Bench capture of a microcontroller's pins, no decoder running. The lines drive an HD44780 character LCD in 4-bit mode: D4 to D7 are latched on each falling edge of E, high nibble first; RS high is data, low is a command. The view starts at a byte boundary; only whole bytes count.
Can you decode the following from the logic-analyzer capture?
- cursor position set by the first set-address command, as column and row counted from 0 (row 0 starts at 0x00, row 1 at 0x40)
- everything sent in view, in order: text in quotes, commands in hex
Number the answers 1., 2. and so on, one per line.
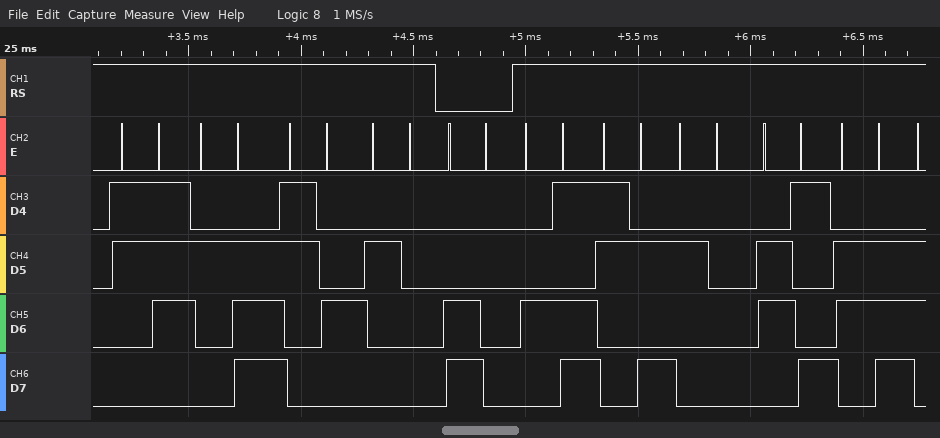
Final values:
1. column 0, row 1
2. "7.4 " 0xC0 "M: in"
